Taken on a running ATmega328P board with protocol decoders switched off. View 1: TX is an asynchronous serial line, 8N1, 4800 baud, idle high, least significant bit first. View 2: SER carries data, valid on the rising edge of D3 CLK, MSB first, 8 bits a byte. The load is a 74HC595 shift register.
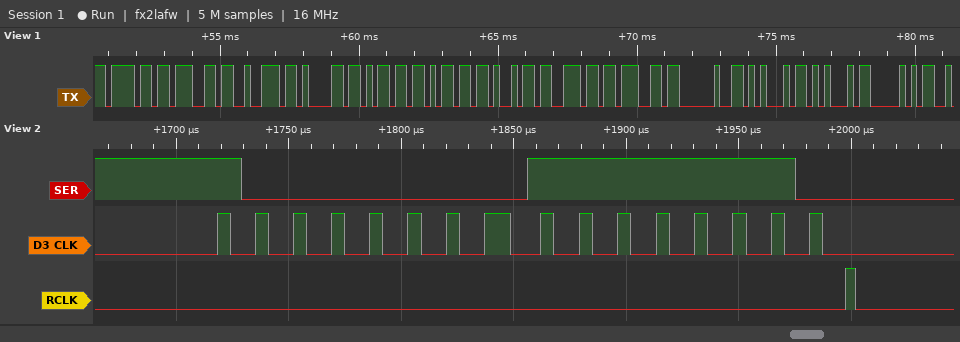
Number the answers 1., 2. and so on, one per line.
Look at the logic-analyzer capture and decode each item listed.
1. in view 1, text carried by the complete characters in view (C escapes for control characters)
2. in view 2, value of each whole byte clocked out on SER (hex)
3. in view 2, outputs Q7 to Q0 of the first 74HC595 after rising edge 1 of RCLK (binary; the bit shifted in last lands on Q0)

1. "ogramming EEP"
2. 80 FE
3. 11111110
